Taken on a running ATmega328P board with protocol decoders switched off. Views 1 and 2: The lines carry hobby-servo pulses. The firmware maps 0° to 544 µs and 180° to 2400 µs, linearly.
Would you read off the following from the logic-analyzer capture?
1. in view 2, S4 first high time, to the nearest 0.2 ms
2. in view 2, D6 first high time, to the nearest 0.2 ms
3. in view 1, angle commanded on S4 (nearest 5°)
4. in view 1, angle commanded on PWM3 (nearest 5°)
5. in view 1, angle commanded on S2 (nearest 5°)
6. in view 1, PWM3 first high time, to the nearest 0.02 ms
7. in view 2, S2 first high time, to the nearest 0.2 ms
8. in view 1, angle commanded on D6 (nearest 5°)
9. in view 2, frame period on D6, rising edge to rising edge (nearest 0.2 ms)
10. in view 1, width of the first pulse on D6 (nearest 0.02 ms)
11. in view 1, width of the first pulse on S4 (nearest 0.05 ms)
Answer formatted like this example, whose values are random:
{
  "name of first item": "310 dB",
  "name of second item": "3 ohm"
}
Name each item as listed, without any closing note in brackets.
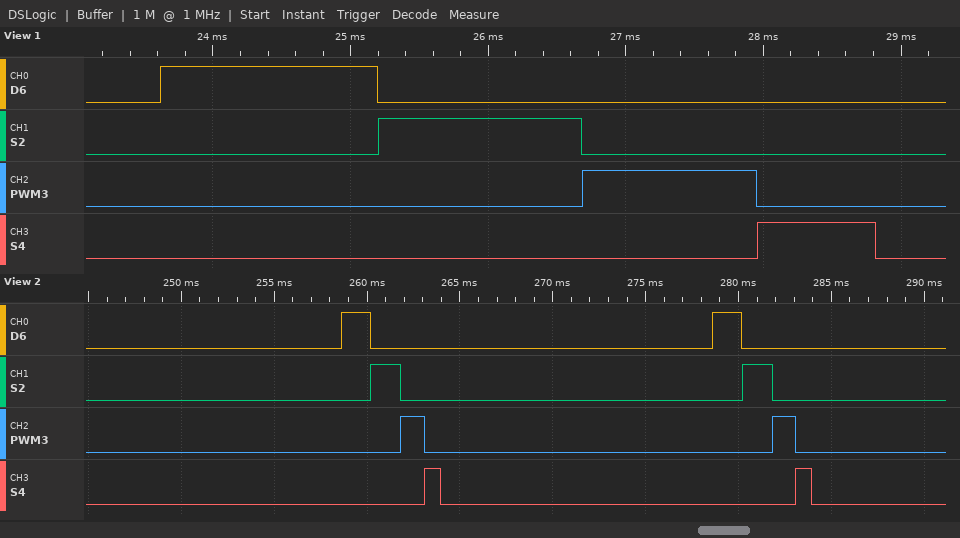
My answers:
{
  "in view 2, S4 first high time, to the nearest 0.2 ms": "0.8 ms",
  "in view 2, D6 first high time, to the nearest 0.2 ms": "1.6 ms",
  "in view 1, angle commanded on S4": "30°",
  "in view 1, angle commanded on PWM3": "70°",
  "in view 1, angle commanded on S2": "90°",
  "in view 1, PWM3 first high time, to the nearest 0.02 ms": "1.26 ms",
  "in view 2, S2 first high time, to the nearest 0.2 ms": "1.6 ms",
  "in view 1, angle commanded on D6": "100°",
  "in view 2, frame period on D6, rising edge to rising edge": "20.0 ms",
  "in view 1, width of the first pulse on D6": "1.58 ms",
  "in view 1, width of the first pulse on S4": "0.85 ms"
}
